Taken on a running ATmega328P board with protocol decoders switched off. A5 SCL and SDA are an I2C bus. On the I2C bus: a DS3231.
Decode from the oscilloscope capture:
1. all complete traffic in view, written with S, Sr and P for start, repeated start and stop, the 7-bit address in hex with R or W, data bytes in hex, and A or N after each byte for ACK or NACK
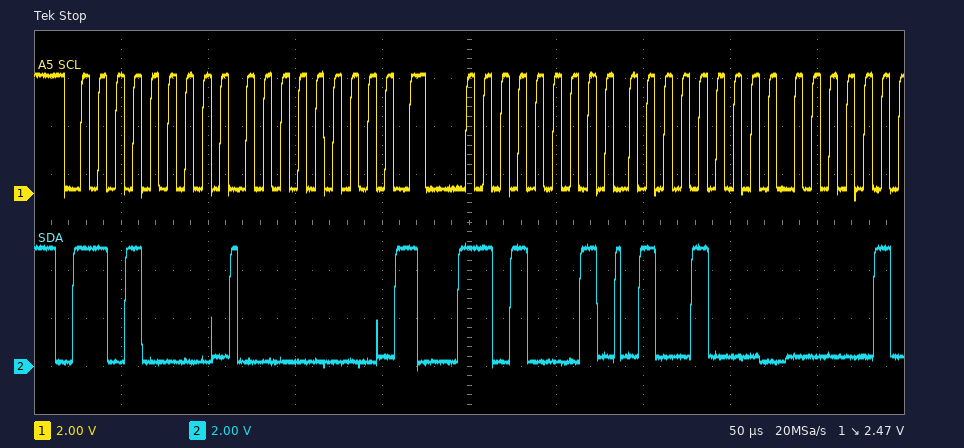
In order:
S 68W A 00 A Sr 68R A 48 A
